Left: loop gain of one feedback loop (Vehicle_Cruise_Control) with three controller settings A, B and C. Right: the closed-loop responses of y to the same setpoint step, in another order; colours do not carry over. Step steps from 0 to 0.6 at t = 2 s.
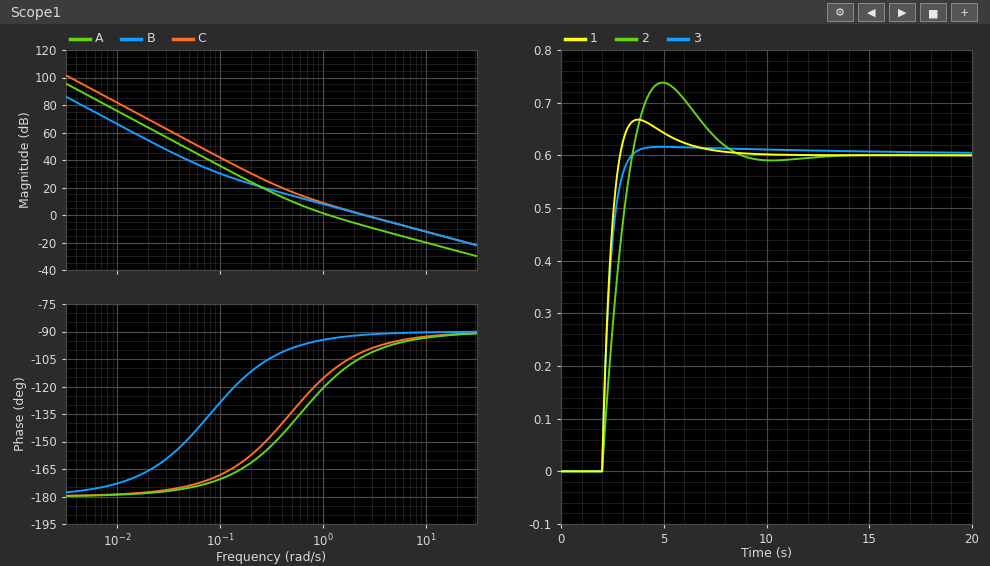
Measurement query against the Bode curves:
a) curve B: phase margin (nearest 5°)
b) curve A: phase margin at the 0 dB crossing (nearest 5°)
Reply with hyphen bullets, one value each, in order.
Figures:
- 90°
- 60°
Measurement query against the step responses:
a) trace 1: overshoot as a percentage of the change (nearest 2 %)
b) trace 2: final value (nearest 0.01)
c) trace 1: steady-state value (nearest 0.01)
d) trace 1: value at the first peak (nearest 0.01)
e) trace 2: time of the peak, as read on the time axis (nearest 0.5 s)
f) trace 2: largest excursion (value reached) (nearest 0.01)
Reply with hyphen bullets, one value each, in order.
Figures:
- 12 %
- 0.60
- 0.60
- 0.67
- 5.0 s
- 0.74
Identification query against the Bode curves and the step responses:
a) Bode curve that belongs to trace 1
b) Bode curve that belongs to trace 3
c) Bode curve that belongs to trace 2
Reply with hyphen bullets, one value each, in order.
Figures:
- C
- B
- A
